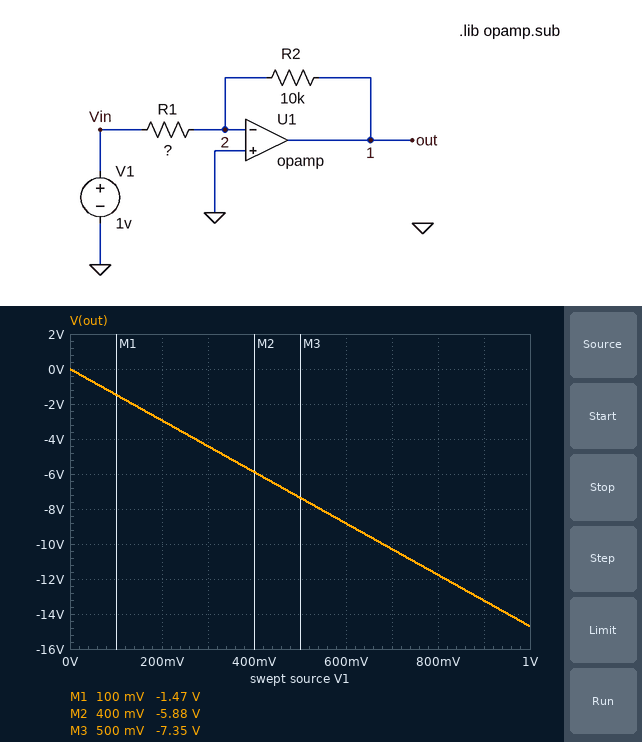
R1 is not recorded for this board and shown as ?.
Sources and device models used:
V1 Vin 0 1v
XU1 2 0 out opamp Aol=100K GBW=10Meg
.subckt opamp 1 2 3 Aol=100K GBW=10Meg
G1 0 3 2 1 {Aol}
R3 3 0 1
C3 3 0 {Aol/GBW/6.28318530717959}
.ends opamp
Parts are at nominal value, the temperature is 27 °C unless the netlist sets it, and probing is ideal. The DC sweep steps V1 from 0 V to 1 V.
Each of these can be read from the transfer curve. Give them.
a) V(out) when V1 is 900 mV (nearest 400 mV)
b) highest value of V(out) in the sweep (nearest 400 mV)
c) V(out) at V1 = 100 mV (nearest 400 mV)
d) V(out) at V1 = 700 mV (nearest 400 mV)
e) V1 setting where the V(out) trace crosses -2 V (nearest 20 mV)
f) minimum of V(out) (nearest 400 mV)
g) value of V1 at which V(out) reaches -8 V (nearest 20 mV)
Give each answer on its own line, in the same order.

-13.2 V
0 V
-1.6 V
-10.4 V
140 mV
-14.8 V
540 mV
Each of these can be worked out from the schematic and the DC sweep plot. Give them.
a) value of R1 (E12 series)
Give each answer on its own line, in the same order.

680 Ω
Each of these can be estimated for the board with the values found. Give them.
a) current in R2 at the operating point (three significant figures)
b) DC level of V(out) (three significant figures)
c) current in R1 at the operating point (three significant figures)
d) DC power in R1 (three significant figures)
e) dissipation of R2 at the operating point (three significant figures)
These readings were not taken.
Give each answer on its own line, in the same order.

1.47 mA
-14.7 V
1.47 mA
1.47 mW
21.6 mW
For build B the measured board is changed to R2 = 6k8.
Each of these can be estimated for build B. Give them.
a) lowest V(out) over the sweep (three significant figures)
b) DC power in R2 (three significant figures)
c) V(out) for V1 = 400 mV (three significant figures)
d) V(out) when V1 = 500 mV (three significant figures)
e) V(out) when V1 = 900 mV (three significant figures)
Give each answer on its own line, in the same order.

-10.0 V
14.7 mW
-4.00 V
-5.00 V
-9.00 V
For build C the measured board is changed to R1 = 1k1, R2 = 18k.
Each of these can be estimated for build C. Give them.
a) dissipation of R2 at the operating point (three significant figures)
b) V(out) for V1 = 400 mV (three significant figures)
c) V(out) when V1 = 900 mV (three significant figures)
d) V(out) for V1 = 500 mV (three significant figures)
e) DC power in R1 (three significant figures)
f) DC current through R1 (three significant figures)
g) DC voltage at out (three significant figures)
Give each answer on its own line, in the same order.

14.9 mW
-6.54 V
-14.7 V
-8.18 V
909 µW
909 µA
-16.4 V
